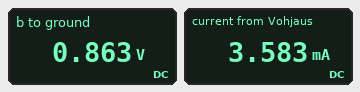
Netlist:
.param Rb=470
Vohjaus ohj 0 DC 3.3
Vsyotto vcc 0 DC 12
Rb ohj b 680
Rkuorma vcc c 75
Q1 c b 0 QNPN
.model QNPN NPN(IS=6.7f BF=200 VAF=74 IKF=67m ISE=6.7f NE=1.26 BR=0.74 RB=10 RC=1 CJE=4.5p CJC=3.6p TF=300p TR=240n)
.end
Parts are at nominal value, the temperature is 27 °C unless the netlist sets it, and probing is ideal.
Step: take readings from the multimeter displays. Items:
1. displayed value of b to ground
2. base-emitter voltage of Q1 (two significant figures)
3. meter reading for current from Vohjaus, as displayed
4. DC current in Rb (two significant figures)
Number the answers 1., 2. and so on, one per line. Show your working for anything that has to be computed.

1. 0.863 V
2. 863 mV = 860 mV
3. 3.583 mA
4. (3.3 V - 863 mV) / 680 Ω = 3.6 mA
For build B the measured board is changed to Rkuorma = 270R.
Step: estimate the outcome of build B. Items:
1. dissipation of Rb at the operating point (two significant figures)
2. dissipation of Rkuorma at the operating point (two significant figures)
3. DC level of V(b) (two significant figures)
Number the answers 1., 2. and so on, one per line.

1. 9.1 mW
2. 520 mW
3. 820 mV
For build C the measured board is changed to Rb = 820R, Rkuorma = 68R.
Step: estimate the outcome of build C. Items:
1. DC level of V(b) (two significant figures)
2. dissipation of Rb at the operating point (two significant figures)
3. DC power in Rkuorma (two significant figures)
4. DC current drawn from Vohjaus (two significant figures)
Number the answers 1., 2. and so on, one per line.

1. 850 mV
2. 7.3 mW
3. 1.5 W
4. 3.0 mA
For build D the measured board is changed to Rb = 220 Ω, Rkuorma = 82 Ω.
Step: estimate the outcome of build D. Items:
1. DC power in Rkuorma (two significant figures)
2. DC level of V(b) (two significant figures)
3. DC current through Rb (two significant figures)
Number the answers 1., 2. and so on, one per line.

1. 1.7 W
2. 930 mV
3. 11 mA
